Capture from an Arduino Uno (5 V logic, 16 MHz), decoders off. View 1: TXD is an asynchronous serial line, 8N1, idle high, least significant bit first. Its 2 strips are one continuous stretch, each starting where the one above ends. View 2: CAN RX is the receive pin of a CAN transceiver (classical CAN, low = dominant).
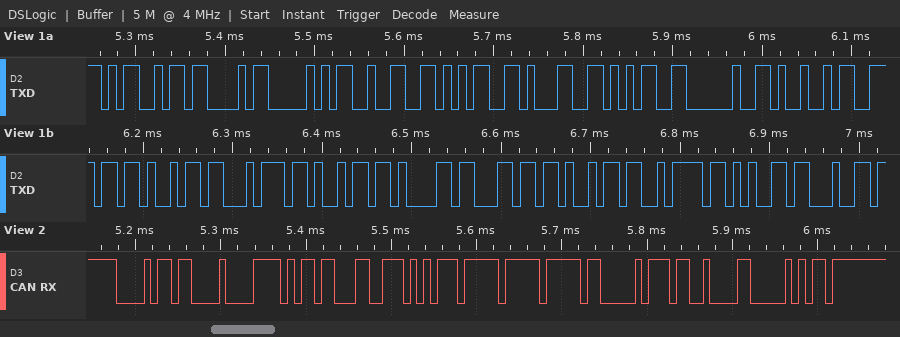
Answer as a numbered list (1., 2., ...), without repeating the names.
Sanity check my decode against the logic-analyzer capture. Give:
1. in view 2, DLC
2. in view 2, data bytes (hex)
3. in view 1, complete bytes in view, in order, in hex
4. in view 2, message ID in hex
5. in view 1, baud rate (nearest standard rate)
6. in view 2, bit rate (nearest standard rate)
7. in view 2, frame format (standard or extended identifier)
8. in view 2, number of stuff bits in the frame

1. 8
2. 7A D8 CE AE FF FF 81 D9
3. 0x4D 0x43 0x50 0x32 0x35 0x31 0x35 0x20 0x49 0x6E 0x69 0x74 0x69 0x61 0x6C 0x69 0x7A 0x65 0x64
4. 0x0B6
5. 115200 baud
6. 125 kbit/s
7. standard
8. 5
